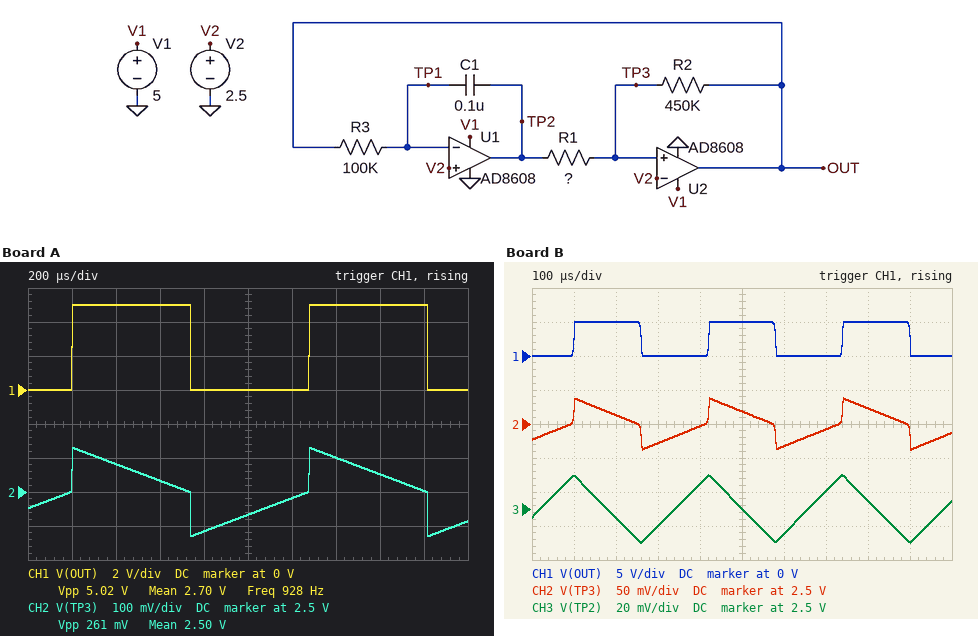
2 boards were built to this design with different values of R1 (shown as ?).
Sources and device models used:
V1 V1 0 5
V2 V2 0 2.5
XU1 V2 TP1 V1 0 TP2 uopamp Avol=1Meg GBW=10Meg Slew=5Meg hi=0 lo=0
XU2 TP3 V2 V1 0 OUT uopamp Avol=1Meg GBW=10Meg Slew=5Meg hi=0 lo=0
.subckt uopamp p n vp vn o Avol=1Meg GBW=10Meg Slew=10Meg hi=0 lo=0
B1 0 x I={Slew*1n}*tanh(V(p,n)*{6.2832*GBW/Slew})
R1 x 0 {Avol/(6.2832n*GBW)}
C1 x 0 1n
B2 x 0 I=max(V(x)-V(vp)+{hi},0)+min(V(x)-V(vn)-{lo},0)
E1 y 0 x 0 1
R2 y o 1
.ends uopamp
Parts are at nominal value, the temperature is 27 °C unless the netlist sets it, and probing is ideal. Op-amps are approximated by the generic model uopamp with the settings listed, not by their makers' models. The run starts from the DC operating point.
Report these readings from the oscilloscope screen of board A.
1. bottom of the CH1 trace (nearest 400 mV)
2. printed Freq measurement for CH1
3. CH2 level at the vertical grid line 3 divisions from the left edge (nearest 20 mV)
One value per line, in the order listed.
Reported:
0 V
928 Hz
2.54 V
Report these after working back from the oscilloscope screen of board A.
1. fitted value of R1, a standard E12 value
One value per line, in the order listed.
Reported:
12 kΩ
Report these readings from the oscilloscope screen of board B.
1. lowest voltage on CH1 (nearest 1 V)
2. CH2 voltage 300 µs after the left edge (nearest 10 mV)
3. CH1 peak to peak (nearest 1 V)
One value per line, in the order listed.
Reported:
0 V
2.47 V
5 V
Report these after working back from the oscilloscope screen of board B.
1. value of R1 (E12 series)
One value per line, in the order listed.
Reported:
3.3 kΩ
